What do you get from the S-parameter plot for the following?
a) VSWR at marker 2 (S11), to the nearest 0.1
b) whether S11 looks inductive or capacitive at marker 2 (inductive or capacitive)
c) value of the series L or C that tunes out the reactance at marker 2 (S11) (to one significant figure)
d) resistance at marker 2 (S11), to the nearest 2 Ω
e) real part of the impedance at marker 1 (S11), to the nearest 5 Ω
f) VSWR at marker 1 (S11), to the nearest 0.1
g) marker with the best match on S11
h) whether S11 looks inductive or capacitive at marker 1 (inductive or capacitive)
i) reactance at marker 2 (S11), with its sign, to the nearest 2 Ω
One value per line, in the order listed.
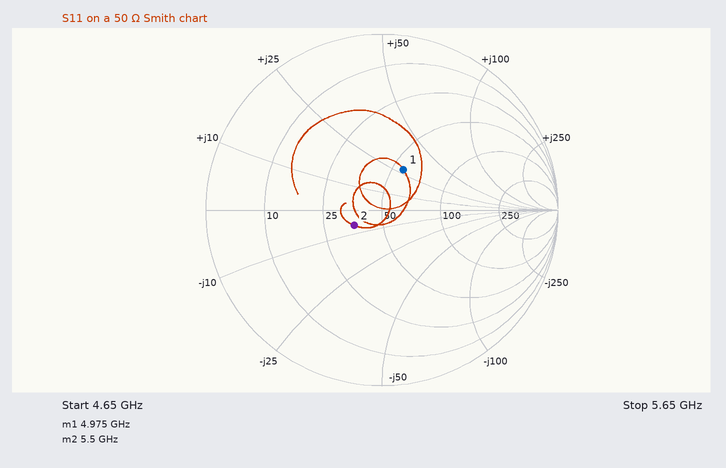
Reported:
1.4
capacitive
200 pH
36 Ω
55 Ω
1.7
marker 2
inductive
-6 Ω
